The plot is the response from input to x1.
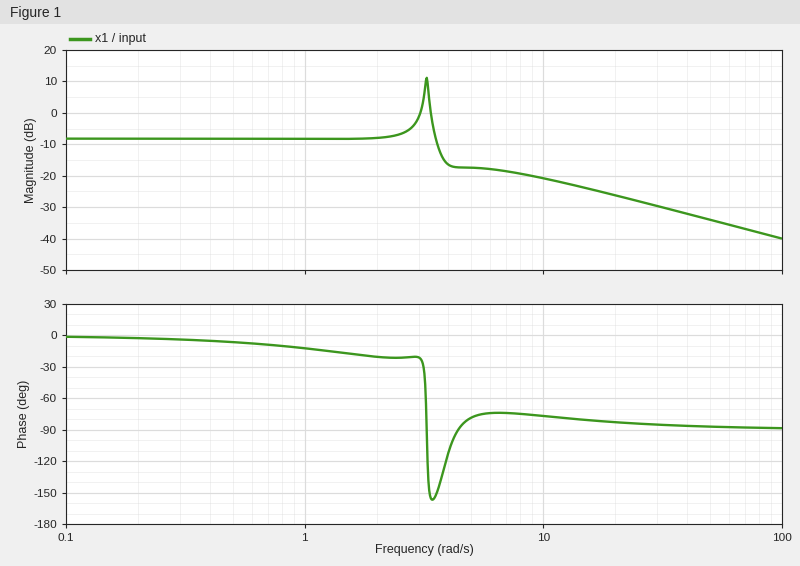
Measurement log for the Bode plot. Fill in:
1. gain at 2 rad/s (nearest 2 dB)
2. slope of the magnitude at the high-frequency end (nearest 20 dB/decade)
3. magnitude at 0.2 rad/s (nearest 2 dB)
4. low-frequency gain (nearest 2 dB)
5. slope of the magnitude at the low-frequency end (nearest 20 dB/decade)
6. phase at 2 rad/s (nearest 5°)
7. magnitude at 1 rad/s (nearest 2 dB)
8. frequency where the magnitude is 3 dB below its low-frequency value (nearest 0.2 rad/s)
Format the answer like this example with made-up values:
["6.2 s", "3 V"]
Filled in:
["-8 dB", "-20 dB/decade", "-8 dB", "-8 dB", "0 dB/decade", "-20°", "-8 dB", "3.6 rad/s"]
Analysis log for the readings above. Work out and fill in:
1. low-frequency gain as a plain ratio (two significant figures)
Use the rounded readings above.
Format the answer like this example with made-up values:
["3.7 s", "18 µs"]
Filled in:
["0.40"]
